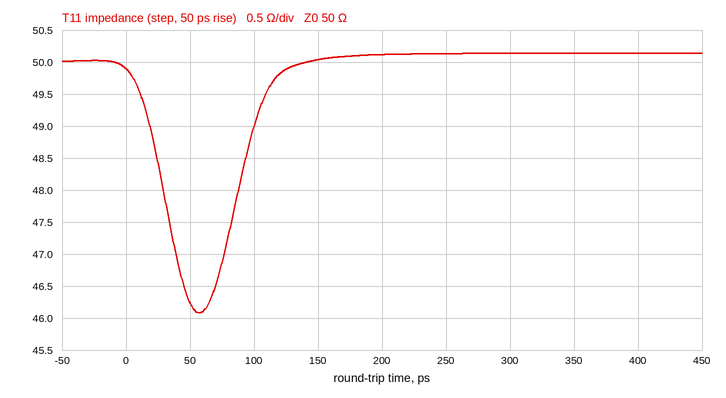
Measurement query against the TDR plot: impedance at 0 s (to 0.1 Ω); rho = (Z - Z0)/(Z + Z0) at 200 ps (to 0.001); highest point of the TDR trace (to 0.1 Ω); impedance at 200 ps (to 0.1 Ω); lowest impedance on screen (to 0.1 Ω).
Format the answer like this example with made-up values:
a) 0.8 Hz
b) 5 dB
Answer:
a) 49.9 Ω
b) +0.001
c) 50.1 Ω
d) 50.1 Ω
e) 46.1 Ω
